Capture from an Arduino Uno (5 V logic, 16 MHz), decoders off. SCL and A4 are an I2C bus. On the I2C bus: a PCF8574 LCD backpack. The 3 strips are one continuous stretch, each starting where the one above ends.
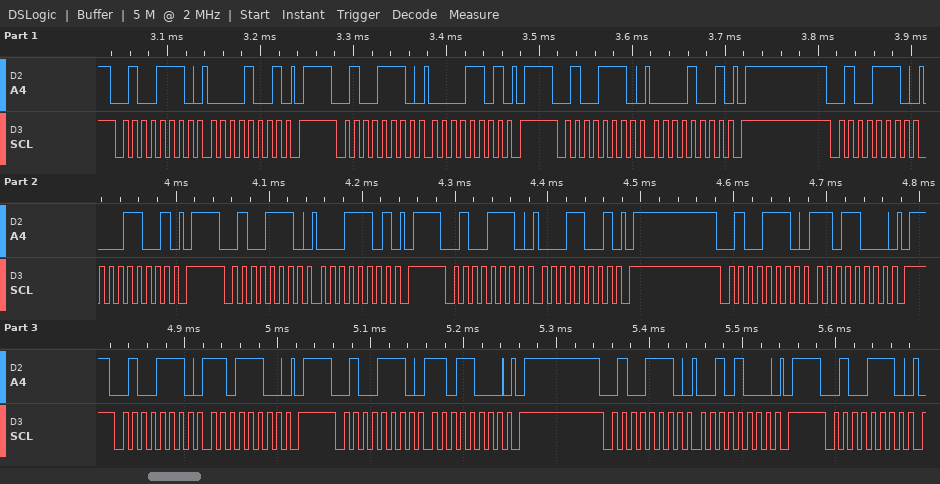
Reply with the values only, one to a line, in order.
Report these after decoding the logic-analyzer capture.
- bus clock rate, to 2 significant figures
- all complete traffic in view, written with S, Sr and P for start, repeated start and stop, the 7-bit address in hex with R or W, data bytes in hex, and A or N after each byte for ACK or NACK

100 kHz
S 27W A 09 A P S 27W A 0D A P S 27W A 09 A P S 27W A 19 A P S 27W A 1D A P S 27W A 19 A P S 27W A D8 A P S 27W A DC A P S 27W A D8 A P S 27W A 28 A P S 27W A
